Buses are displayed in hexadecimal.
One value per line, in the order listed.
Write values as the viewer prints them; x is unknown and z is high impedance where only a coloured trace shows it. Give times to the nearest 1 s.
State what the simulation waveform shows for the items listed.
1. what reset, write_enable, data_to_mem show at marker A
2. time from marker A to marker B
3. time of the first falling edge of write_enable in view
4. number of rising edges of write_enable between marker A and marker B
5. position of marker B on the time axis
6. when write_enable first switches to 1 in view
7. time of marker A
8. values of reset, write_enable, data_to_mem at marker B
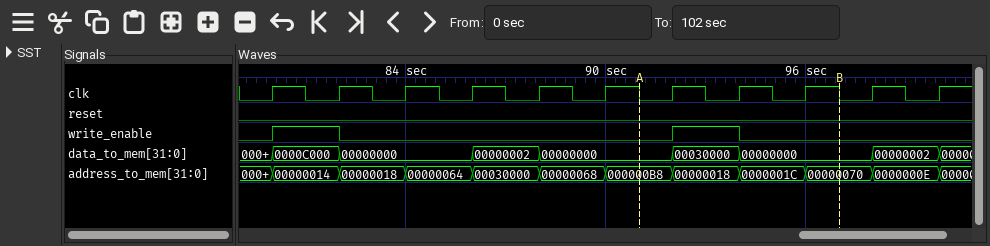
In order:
reset=0, write_enable=0, data_to_mem=00000000
6 s
82 s
1
97 s
80 s
91 s
reset=0, write_enable=0, data_to_mem=00000000
